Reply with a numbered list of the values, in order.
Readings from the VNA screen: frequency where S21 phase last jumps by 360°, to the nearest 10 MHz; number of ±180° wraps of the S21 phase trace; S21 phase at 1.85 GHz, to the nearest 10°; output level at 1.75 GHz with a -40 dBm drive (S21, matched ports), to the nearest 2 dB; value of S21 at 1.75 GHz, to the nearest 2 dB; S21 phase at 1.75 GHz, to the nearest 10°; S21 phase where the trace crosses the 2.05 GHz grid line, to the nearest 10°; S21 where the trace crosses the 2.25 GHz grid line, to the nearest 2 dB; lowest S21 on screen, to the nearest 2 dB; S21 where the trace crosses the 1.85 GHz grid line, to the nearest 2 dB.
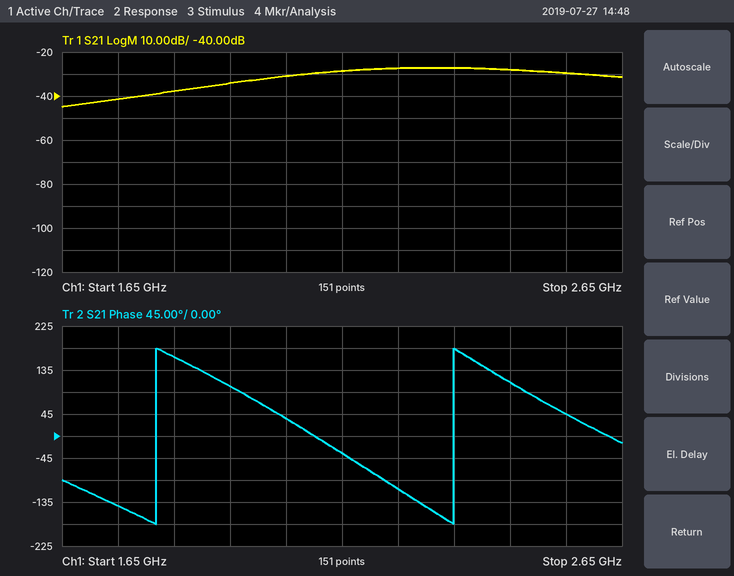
1. 2.35 GHz
2. 2
3. 160°
4. -82 dBm
5. -42 dB
6. -140°
7. 40°
8. -28 dB
9. -44 dB
10. -38 dB
